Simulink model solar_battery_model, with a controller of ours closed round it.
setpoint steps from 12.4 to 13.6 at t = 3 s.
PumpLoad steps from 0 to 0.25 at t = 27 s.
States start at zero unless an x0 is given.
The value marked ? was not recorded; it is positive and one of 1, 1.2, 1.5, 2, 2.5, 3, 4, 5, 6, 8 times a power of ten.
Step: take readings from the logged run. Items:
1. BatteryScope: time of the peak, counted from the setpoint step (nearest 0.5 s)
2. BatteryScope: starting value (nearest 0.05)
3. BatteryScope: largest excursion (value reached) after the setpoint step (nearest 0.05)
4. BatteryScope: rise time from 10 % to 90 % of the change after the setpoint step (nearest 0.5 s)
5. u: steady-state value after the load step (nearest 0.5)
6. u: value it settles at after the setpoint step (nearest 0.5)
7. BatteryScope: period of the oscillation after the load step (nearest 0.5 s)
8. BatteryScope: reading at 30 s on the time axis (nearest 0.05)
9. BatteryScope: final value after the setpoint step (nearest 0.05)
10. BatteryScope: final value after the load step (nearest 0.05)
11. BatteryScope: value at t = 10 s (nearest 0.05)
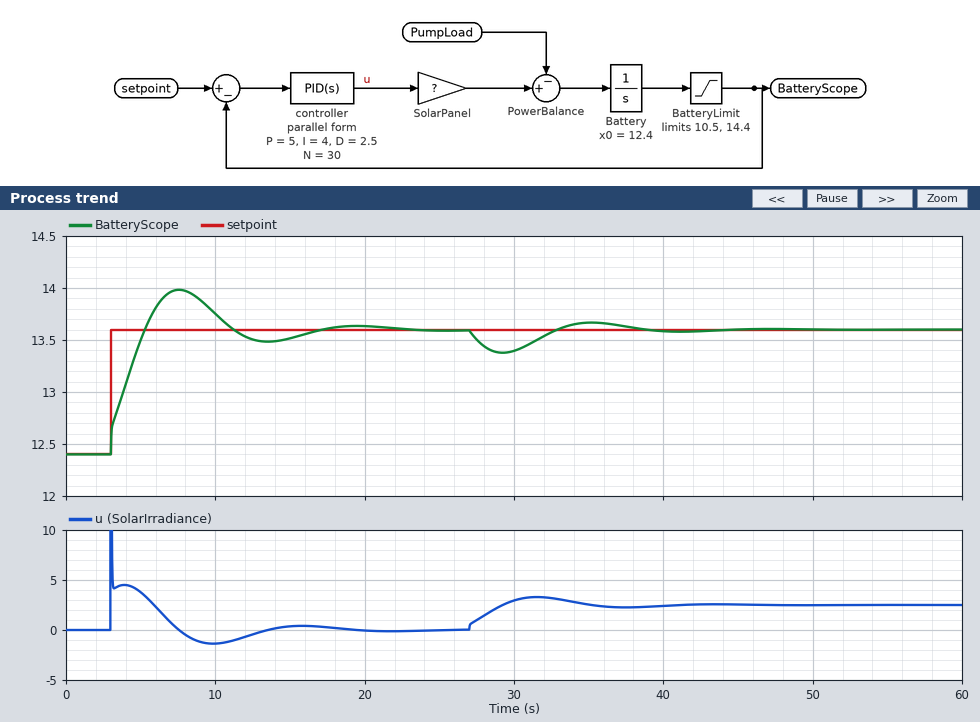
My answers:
4.5 s
12.40
14.00
2.0 s
2.5
0.0
12.0 s
13.40
13.60
13.60
13.75
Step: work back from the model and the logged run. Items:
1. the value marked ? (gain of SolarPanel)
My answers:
0.1
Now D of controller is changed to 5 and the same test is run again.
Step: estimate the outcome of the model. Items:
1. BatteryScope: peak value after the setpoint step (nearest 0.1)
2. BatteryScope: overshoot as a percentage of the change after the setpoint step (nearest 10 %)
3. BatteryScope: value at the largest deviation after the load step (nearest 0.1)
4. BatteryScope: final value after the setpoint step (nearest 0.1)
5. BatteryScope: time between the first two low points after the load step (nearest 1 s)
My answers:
13.9
30 %
13.4
13.6
13 s
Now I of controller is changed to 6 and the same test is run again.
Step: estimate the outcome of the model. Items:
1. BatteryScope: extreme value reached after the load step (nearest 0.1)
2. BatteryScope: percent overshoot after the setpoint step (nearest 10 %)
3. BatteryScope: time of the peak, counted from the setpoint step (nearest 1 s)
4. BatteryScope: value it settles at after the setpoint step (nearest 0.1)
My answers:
13.4
40 %
4 s
13.6
